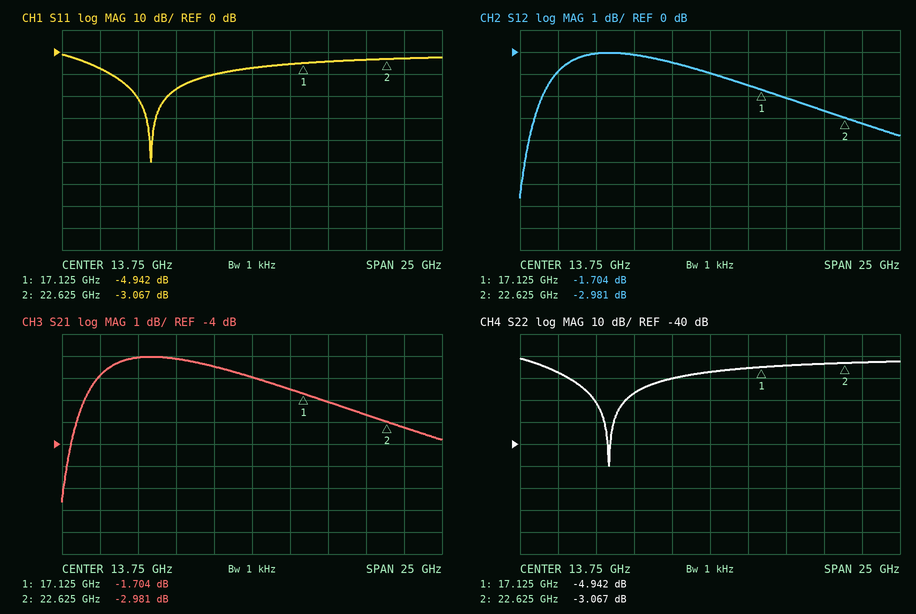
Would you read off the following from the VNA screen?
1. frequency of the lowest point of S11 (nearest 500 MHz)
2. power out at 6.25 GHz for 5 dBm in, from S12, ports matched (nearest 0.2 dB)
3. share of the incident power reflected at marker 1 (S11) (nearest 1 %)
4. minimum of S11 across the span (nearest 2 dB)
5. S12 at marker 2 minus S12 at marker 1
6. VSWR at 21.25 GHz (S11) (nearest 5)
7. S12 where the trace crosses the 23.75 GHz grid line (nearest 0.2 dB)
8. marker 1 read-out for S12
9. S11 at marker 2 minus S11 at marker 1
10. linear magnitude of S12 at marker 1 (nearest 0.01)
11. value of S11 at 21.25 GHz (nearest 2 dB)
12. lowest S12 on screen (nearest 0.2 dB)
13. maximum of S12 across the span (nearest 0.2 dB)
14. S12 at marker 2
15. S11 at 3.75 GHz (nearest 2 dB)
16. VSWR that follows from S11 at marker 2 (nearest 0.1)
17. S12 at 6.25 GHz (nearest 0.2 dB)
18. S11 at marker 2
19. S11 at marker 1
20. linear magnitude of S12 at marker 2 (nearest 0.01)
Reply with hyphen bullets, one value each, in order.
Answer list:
- 7.0 GHz
- 5.0 dBm
- 32 %
- -50 dB
- -1.277 dB
- 5
- -3.2 dB
- -1.704 dB
- 1.875 dB
- 0.82
- -4 dB
- -6.6 dB
- 0.0 dB
- -2.981 dB
- -8 dB
- 5.7
- 0.0 dB
- -3.067 dB
- -4.942 dB
- 0.71
